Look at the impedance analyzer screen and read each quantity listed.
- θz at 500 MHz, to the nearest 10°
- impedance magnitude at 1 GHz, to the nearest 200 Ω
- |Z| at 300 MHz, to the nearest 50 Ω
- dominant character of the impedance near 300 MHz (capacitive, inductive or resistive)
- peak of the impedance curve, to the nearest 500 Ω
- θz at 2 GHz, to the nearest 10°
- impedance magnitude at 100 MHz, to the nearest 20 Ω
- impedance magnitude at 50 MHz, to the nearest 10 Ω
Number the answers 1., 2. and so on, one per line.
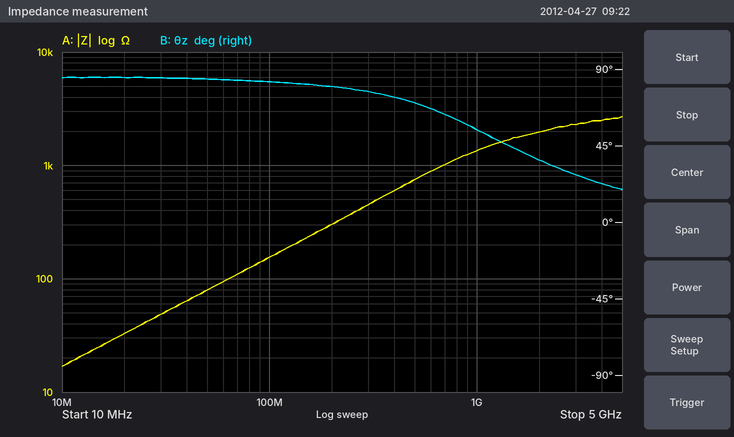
1. 70°
2. 1.4 kΩ
3. 450 Ω
4. inductive
5. 2.5 kΩ
6. 40°
7. 160 Ω
8. 80 Ω
